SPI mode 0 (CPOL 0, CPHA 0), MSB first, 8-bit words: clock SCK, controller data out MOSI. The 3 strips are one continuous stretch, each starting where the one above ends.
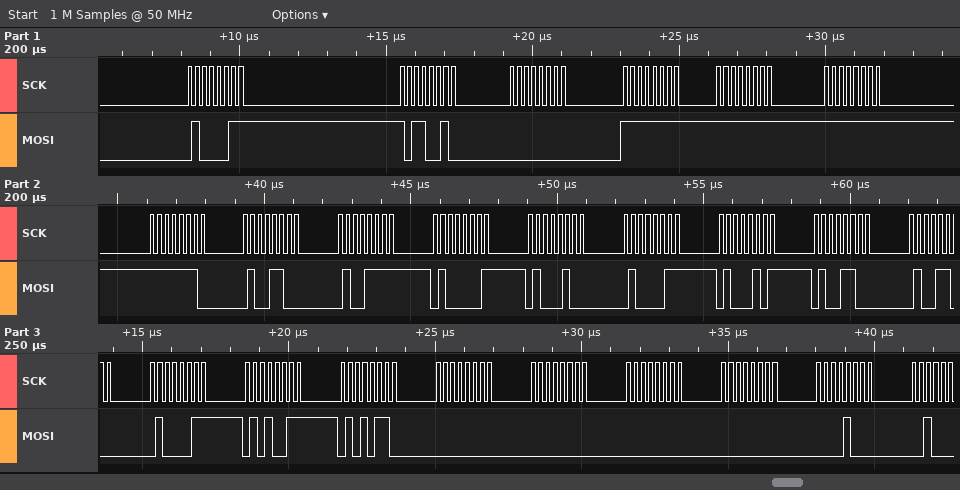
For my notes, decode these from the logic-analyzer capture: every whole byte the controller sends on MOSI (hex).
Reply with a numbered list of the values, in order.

1. 43 B2 00 FF FF FF FE 4C 4F 41 44 43 45 4C 4C 43 53 56 00 00 00 00 08
